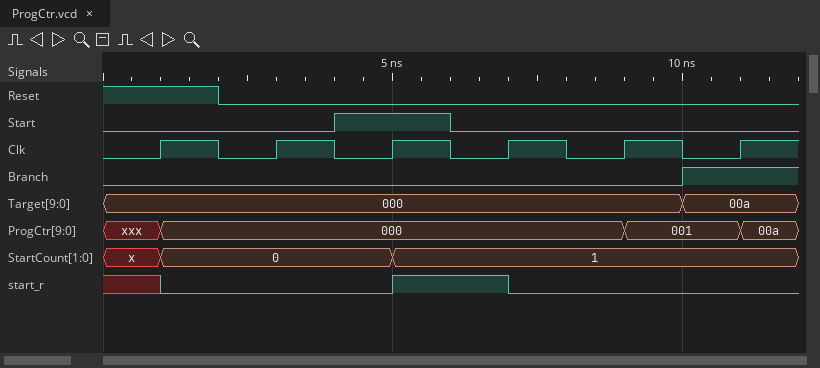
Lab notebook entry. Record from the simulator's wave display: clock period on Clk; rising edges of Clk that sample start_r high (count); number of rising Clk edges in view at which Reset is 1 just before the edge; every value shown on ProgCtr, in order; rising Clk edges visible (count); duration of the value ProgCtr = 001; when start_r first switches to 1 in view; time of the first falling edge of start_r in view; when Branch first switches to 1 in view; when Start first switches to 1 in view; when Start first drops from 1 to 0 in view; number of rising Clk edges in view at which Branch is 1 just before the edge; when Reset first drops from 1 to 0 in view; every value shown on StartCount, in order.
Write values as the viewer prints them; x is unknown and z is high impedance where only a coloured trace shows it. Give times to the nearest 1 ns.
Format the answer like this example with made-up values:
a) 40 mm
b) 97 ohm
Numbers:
a) 2 ns
b) 1
c) 1
d) xxx, 000, 001, 00a
e) 6
f) 2 ns
g) 5 ns
h) 7 ns
i) 10 ns
j) 4 ns
k) 6 ns
l) 1
m) 2 ns
n) x, 0, 1
